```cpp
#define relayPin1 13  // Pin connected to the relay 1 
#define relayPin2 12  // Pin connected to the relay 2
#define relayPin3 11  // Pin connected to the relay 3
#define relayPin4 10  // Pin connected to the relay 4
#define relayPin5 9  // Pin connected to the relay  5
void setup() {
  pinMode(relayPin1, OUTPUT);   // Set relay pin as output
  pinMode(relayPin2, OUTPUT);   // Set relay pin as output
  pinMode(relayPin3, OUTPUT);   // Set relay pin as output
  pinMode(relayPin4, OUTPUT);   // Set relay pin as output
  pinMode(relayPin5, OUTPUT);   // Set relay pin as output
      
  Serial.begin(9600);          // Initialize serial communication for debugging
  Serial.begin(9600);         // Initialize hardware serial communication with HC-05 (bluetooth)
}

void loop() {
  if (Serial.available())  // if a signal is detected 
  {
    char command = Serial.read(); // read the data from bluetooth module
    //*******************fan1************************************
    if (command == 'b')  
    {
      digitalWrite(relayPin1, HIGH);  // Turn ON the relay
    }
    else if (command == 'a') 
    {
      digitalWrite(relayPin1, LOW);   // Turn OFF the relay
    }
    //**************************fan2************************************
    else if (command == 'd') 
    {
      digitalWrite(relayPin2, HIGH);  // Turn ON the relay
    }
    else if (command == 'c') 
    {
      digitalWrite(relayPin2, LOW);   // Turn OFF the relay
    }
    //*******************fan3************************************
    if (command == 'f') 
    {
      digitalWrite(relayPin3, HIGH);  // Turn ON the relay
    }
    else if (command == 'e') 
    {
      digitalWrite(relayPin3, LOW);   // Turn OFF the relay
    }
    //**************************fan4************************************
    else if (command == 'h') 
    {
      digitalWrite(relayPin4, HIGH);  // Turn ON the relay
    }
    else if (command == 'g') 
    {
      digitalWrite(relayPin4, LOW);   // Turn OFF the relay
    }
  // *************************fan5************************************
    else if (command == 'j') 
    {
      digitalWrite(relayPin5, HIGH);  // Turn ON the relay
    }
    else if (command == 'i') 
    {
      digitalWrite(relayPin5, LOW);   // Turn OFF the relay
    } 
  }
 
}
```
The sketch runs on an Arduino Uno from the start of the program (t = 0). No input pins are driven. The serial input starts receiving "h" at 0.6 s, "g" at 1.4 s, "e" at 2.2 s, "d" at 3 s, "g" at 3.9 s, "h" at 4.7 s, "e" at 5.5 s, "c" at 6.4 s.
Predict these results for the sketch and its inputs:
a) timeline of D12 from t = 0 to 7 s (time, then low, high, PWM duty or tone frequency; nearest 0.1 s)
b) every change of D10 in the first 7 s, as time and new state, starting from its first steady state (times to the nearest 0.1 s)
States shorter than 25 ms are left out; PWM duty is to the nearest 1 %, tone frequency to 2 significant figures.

0 s low; 3 s high; 6.4 s low
0 s low; 0.6 s high; 1.4 s low; 4.7 s high
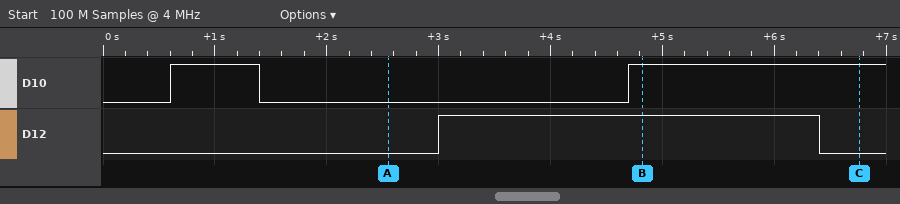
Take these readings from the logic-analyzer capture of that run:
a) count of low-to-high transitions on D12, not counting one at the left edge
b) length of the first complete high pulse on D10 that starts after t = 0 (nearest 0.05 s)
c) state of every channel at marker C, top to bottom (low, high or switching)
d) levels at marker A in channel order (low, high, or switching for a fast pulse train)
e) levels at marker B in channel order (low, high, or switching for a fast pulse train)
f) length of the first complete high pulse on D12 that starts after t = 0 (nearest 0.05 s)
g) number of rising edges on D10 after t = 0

1
0.80 s
D10 high, D12 low
D10 low, D12 low
D10 high, D12 high
3.40 s
2
